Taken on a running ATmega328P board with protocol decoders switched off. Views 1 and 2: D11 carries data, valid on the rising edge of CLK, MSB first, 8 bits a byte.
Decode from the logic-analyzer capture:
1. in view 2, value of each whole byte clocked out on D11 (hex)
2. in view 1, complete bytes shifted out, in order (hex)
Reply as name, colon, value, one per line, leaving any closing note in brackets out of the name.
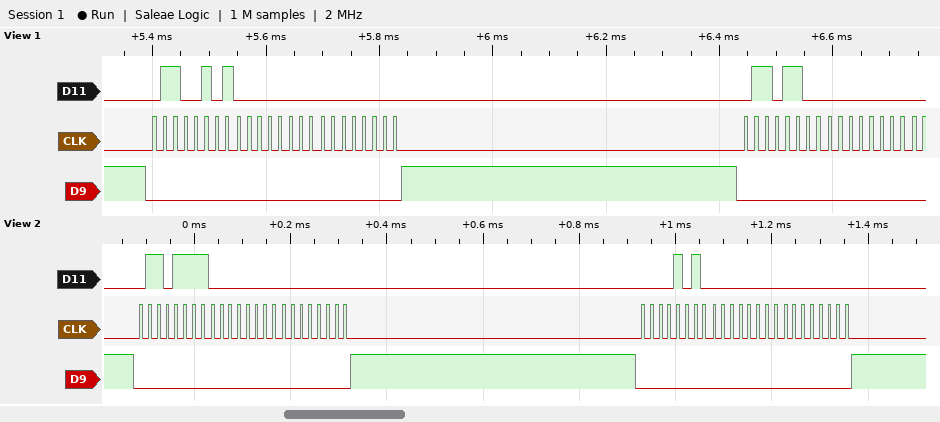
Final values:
in view 2, value of each whole byte clocked out on D11: 0x6F 0x00 0x00 0x0A 0x00 0x00
in view 1, complete bytes shifted out, in order: 0x65 0x00 0x00 0x6C 0x00
